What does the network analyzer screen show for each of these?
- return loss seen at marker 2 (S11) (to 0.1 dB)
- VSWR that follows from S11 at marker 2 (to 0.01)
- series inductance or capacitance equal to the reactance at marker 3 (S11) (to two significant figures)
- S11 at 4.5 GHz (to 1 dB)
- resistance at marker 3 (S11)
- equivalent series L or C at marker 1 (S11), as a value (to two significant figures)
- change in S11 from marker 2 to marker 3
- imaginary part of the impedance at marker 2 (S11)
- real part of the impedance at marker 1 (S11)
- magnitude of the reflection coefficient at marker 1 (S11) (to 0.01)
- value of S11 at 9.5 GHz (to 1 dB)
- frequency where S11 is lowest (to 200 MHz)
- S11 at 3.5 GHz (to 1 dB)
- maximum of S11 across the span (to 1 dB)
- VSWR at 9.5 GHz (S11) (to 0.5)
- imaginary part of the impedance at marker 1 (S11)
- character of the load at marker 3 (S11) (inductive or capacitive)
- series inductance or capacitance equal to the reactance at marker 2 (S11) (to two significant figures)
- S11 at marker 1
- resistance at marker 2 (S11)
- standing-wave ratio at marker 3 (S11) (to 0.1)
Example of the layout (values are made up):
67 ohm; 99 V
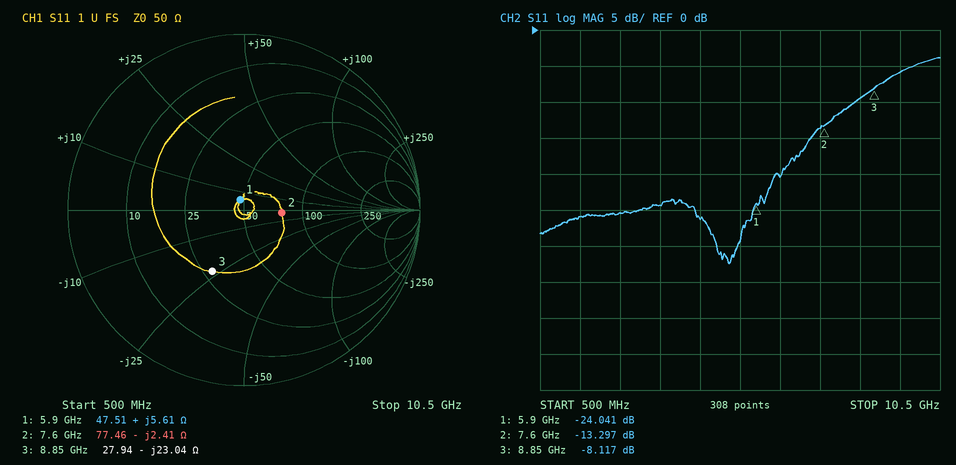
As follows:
13.3 dB; 1.55; 780 fF; -26 dB; 27.94 Ω; 150 pH; 5.180 dB; -2.41 Ω; 47.51 Ω; 0.06; -6 dB; 5.2 GHz; -24 dB; -4 dB; 3.0; +5.61 Ω; capacitive; 8.7 pF; -24.041 dB; 77.46 Ω; 2.3
